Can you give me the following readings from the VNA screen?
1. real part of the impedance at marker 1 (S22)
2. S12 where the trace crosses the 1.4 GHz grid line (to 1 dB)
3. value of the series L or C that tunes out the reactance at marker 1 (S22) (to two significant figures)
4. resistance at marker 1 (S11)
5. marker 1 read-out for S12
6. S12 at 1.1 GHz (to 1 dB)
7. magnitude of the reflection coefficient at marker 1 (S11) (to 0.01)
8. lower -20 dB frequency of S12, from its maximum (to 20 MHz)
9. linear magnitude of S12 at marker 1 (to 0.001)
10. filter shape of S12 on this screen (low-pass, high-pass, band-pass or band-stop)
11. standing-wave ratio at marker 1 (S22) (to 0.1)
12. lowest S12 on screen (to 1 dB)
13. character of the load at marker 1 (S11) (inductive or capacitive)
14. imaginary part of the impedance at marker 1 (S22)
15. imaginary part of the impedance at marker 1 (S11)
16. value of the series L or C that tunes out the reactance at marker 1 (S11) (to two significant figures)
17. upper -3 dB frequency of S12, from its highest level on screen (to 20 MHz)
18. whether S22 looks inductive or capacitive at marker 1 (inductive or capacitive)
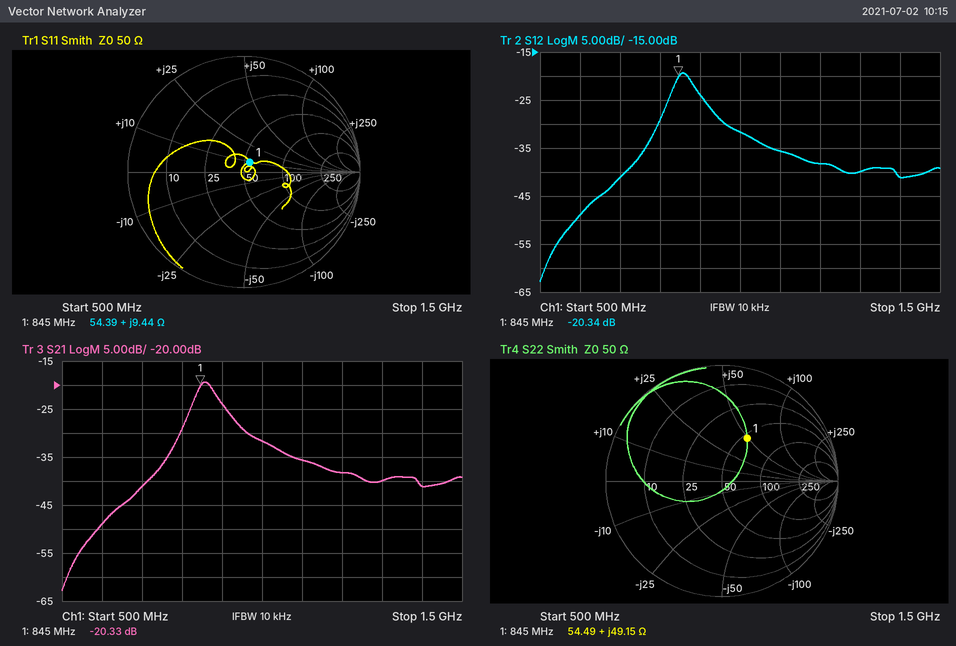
54.49 Ω
-41 dB
3.8 pF
54.39 Ω
-20.34 dB
-36 dB
0.10
720 MHz
0.096
band-pass
2.5
-63 dB
inductive
+49.15 Ω
+9.44 Ω
20 pF
880 MHz
inductive
